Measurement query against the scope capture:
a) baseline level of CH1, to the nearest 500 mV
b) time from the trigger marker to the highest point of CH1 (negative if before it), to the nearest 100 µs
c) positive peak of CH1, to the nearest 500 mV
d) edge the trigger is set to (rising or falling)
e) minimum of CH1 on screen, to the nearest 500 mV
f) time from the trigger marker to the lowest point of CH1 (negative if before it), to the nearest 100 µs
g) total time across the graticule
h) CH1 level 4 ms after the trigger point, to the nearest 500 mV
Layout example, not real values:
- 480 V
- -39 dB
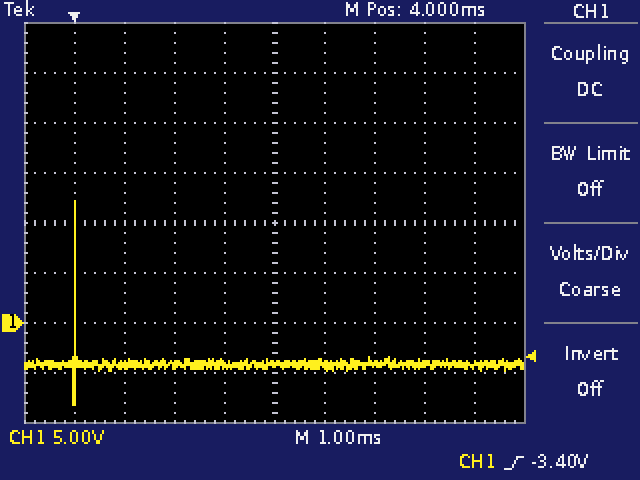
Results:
- -4.0 V
- 0.0 ms
- 12.0 V
- rising
- -8.0 V
- 0.0 ms
- 10 ms
- -4.0 V
